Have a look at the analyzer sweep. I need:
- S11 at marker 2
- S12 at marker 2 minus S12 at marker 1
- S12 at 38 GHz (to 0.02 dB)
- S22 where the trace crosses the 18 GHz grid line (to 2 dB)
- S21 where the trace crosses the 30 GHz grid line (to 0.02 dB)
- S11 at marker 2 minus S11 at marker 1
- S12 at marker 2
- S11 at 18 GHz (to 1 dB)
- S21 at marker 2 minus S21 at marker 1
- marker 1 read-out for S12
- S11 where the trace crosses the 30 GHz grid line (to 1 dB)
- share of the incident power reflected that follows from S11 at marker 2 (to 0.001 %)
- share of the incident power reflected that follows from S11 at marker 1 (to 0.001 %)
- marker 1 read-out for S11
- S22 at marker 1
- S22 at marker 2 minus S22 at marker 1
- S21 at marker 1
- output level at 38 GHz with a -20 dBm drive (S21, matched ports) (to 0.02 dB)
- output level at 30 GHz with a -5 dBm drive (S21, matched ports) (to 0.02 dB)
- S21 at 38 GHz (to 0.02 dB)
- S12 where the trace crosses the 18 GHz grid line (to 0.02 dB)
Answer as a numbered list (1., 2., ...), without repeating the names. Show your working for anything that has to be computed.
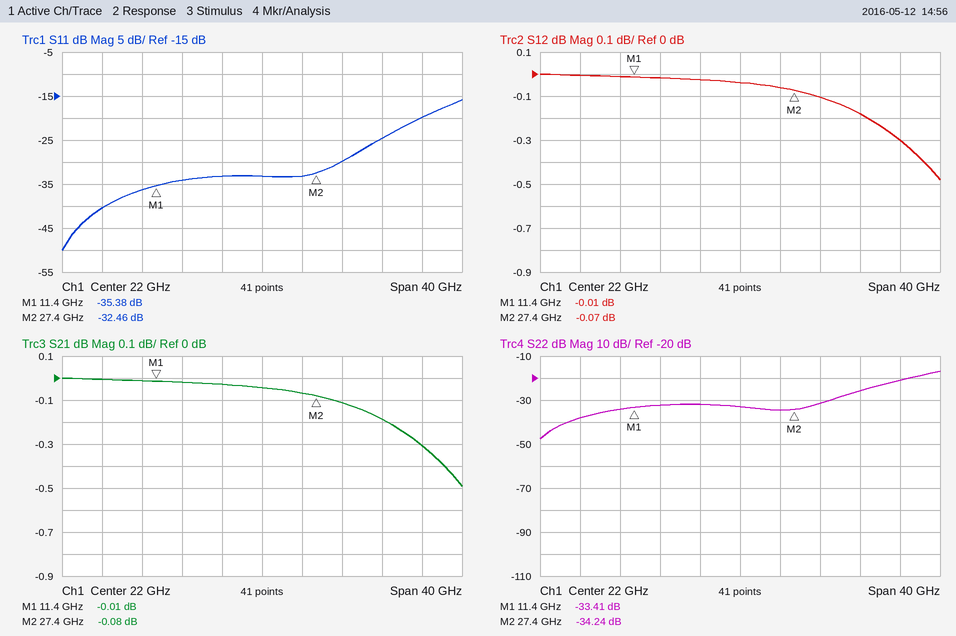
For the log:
1. -32.46 dB
2. -0.07 − (-0.01) = -0.06 dB
3. -0.30 dB
4. -32 dB
5. -0.12 dB
6. -32.46 − (-35.38) = 2.92 dB
7. -0.07 dB
8. -33 dB
9. -0.08 − (-0.01) = -0.07 dB
10. -0.01 dB
11. -30 dB
12. 10^(-32.46/10) ≈ 0.057 %
13. 10^(-35.38/10) ≈ 0.029 %
14. -35.38 dB
15. -33.41 dB
16. -34.24 − (-33.41) = -0.83 dB
17. -0.01 dB
18. -20 dBm + (-0.30 dB) = -20.30 dBm
19. -5 dBm + (-0.12 dB) = -5.12 dBm
20. -0.30 dB
21. -0.02 dB
